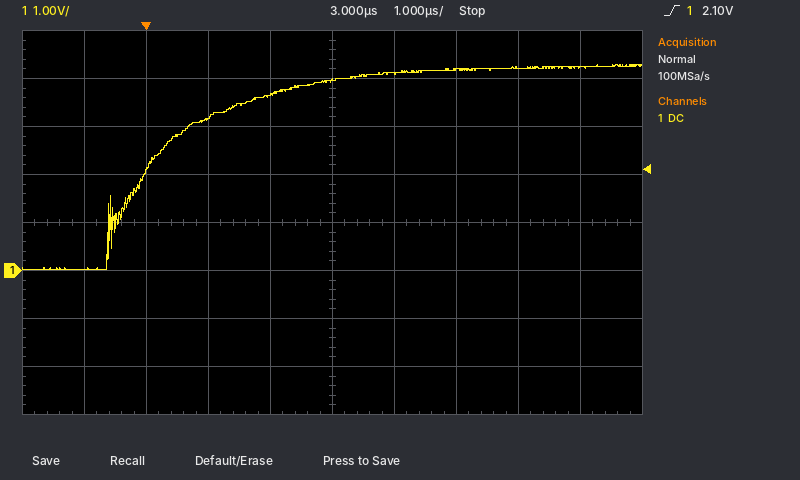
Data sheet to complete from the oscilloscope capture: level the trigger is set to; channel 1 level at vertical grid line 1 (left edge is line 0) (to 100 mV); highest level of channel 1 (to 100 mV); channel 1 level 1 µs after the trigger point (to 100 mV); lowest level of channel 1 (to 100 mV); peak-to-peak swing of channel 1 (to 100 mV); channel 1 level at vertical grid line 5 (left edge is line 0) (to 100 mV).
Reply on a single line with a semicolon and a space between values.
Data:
2.10 V; 0.0 V; 4.3 V; 3.2 V; 0.0 V; 4.3 V; 4.0 V
